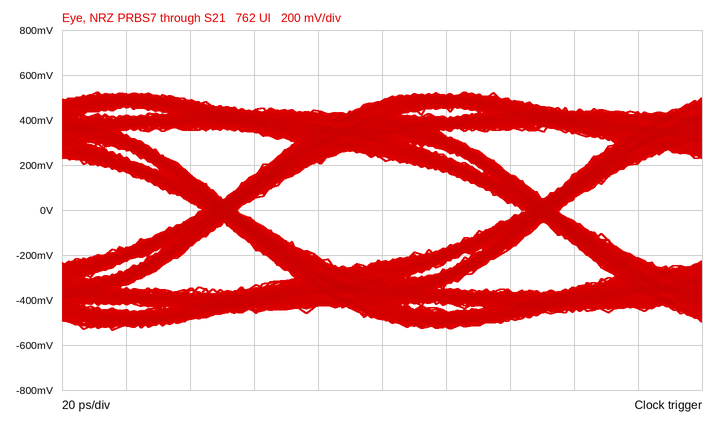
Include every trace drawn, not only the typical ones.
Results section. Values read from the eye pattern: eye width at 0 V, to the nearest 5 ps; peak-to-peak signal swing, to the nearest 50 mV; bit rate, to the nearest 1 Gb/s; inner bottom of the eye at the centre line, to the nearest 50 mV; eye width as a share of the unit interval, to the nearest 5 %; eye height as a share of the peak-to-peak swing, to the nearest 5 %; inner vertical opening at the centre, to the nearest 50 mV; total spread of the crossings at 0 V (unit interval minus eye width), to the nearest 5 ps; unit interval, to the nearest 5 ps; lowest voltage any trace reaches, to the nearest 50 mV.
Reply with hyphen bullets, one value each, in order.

- 90 ps
- 1.05 V
- 10 Gb/s
- -250 mV
- 90 %
- 45 %
- 450 mV
- 10 ps
- 100 ps
- -550 mV
